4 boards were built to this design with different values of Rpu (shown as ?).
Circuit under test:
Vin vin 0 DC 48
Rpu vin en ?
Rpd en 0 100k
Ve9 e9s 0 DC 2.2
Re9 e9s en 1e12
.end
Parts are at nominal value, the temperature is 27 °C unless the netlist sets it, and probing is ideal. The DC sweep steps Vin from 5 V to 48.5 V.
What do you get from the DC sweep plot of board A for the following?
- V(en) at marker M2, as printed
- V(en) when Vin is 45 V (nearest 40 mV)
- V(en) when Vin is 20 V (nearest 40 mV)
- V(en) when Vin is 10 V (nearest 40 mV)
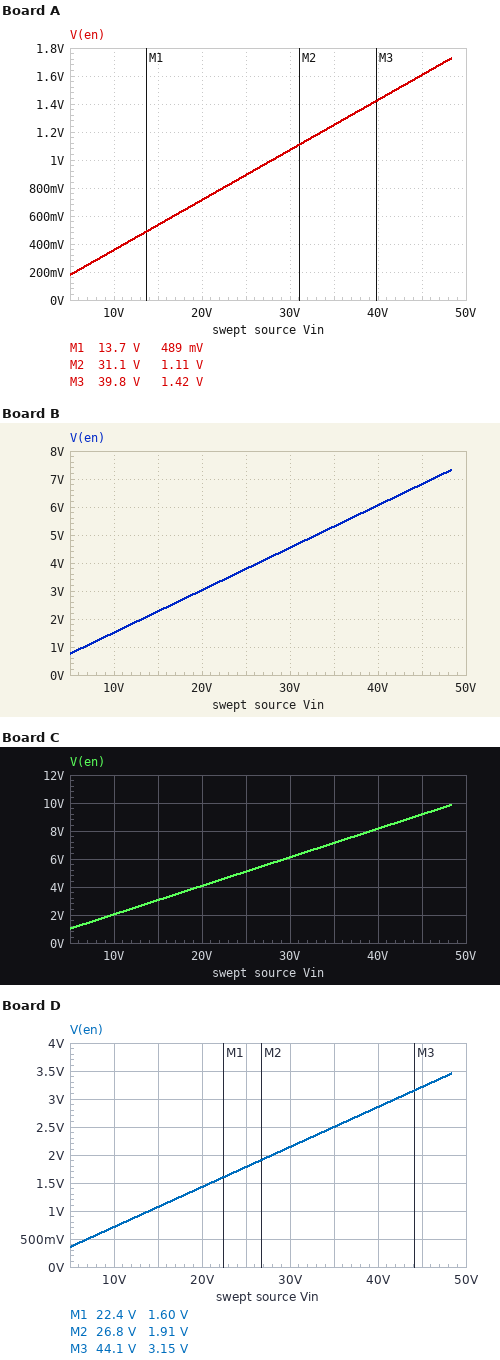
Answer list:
1.11 V
1.60 V
720 mV
360 mV
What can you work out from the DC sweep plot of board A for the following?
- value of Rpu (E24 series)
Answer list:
2.7 MΩ
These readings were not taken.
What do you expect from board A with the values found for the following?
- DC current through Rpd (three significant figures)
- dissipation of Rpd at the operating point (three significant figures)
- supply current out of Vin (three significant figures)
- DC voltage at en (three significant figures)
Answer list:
17.1 µA
29.4 µW
17.1 µA
1.71 V
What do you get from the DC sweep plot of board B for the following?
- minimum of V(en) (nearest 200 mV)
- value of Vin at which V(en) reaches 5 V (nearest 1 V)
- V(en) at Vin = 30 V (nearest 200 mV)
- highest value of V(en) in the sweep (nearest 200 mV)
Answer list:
800 mV
33 V
4.6 V
7.4 V
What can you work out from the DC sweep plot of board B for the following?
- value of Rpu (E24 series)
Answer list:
560 kΩ
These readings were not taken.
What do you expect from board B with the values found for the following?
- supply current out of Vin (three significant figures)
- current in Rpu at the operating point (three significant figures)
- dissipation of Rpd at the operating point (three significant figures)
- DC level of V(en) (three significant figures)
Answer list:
72.7 µA
72.7 µA
529 µW
7.27 V
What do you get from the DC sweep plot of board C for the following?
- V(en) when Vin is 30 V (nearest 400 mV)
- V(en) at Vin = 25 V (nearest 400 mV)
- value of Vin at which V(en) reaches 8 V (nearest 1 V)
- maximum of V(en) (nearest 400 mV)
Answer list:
6.0 V
5.2 V
39 V
10.0 V
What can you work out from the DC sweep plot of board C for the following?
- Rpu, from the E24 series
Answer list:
390 kΩ
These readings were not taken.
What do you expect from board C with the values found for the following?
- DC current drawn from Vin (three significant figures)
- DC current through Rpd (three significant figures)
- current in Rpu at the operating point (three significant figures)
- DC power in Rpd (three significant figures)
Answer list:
98.0 µA
98.0 µA
98.0 µA
960 µW
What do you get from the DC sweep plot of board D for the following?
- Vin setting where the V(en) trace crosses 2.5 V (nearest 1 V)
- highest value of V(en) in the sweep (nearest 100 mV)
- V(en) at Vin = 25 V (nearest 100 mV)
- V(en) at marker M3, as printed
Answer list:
35 V
3.5 V
1.8 V
3.15 V
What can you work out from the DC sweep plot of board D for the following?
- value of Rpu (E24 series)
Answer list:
1.3 MΩ
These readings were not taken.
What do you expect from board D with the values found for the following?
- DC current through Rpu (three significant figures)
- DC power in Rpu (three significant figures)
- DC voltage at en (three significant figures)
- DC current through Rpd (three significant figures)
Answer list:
34.3 µA
1.53 mW
3.43 V
34.3 µA
